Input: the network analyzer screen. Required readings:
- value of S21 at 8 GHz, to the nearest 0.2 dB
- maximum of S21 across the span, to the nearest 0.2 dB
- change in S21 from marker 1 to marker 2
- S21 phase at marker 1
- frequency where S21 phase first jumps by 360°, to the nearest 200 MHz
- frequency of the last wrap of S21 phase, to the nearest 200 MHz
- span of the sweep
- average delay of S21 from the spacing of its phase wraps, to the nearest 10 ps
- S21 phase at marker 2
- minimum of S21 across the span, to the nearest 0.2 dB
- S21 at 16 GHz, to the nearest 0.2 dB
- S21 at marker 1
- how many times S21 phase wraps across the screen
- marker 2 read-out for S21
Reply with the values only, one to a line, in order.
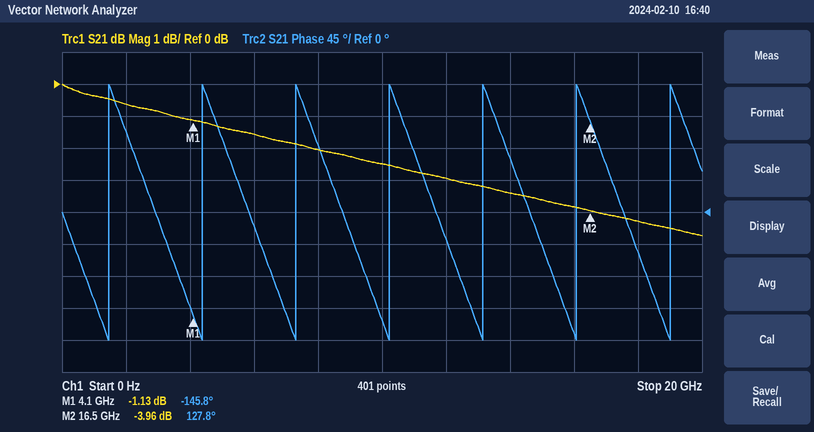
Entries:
-2.0 dB
0.0 dB
-2.83 dB
-145.8°
1.4 GHz
19.0 GHz
20 GHz
340 ps
127.8°
-4.8 dB
-3.8 dB
-1.13 dB
7
-3.96 dB
